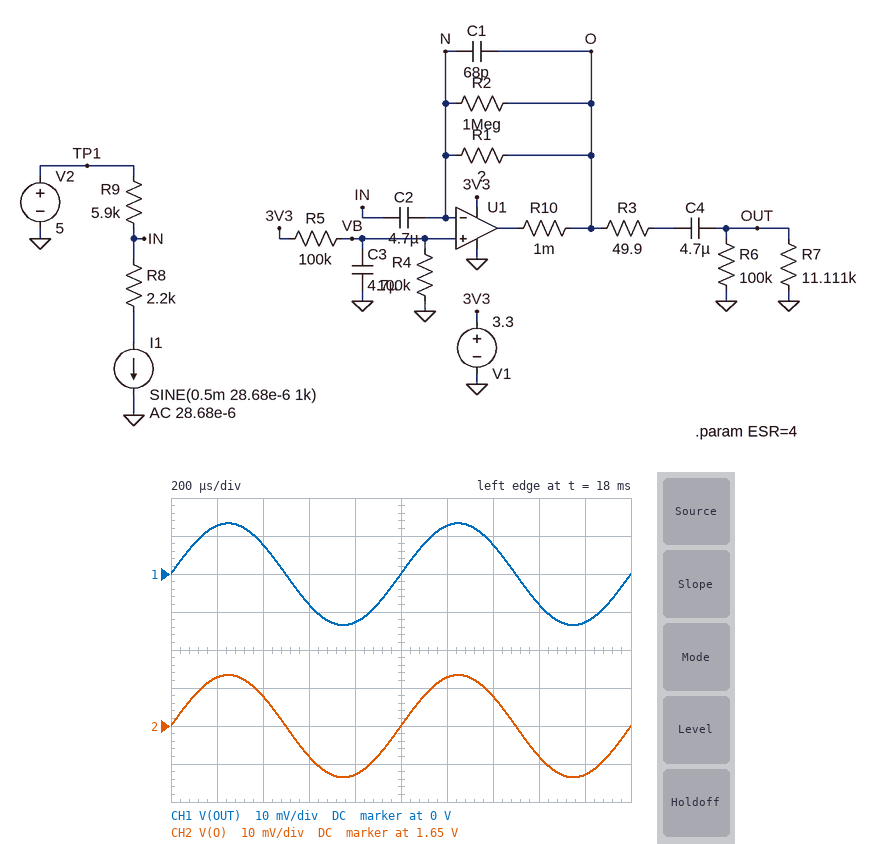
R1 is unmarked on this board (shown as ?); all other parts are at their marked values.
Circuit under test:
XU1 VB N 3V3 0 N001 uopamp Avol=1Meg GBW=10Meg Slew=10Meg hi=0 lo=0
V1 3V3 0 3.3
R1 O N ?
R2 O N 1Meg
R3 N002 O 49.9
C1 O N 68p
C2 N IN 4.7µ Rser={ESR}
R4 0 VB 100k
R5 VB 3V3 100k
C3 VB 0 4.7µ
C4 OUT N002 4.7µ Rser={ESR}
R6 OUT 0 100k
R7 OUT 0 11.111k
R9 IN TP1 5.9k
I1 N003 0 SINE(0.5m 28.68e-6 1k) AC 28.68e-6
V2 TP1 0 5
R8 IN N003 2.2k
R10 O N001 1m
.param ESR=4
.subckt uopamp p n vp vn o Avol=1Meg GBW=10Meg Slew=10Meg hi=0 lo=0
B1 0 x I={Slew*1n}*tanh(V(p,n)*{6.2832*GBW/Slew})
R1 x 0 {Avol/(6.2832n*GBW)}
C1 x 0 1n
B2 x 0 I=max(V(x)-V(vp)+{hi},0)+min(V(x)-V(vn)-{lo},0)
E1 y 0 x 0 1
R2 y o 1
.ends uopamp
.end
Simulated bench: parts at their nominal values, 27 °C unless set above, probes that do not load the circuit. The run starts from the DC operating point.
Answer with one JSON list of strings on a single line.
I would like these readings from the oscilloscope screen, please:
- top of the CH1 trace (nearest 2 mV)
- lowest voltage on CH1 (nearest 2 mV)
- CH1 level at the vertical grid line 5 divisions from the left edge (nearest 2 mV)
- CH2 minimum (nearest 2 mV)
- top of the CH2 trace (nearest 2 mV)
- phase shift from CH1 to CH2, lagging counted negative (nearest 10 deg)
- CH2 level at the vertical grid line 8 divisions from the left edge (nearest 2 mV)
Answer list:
["14 mV", "-14 mV", "0 V", "1.636 V", "1.664 V", "0 deg", "1.642 V"]
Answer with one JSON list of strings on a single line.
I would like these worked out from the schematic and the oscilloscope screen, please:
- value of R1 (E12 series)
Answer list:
["470 Ω"]
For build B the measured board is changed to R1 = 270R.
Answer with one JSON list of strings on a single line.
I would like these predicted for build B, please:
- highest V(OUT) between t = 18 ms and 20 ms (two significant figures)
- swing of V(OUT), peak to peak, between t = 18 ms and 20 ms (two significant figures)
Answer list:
["7.7 mV", "15 mV"]
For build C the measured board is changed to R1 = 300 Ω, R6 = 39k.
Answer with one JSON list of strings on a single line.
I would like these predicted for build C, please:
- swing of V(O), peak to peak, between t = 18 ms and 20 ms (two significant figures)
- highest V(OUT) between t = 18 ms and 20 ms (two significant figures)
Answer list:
["17 mV", "8.5 mV"]
